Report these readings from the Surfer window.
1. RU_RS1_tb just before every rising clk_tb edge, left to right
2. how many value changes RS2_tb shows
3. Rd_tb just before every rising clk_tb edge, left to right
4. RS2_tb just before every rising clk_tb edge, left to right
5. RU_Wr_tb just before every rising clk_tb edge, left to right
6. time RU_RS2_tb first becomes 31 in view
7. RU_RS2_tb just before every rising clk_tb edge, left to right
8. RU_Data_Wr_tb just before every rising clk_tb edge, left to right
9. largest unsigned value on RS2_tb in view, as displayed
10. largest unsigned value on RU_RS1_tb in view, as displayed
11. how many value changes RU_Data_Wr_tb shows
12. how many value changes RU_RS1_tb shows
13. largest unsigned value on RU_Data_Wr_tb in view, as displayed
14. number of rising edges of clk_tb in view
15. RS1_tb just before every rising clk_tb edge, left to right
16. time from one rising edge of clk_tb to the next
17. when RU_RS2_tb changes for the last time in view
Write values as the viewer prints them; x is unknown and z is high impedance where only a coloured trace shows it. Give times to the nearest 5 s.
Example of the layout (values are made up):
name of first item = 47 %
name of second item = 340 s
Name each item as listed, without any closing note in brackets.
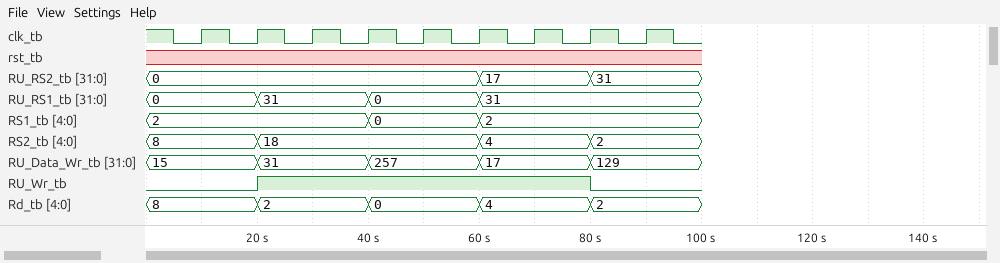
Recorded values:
RU_RS1_tb just before every rising clk_tb edge, left to right = 0, 0, 31, 31, 0, 0, 31, 31, 31
how many value changes RS2_tb shows = 3
Rd_tb just before every rising clk_tb edge, left to right = 8, 8, 2, 2, 0, 0, 4, 4, 2
RS2_tb just before every rising clk_tb edge, left to right = 8, 8, 18, 18, 18, 18, 4, 4, 2
RU_Wr_tb just before every rising clk_tb edge, left to right = 0 0 1 1 1 1 1 1 0
time RU_RS2_tb first becomes 31 in view = 80 s
RU_RS2_tb just before every rising clk_tb edge, left to right = 0, 0, 0, 0, 0, 0, 17, 17, 31
RU_Data_Wr_tb just before every rising clk_tb edge, left to right = 15, 15, 31, 31, 257, 257, 17, 17, 129
largest unsigned value on RS2_tb in view, as displayed = 18
largest unsigned value on RU_RS1_tb in view, as displayed = 31
how many value changes RU_Data_Wr_tb shows = 4
how many value changes RU_RS1_tb shows = 3
largest unsigned value on RU_Data_Wr_tb in view, as displayed = 257
number of rising edges of clk_tb in view = 9
RS1_tb just before every rising clk_tb edge, left to right = 2, 2, 2, 2, 0, 0, 2, 2, 2
time from one rising edge of clk_tb to the next = 10 s
when RU_RS2_tb changes for the last time in view = 80 s
